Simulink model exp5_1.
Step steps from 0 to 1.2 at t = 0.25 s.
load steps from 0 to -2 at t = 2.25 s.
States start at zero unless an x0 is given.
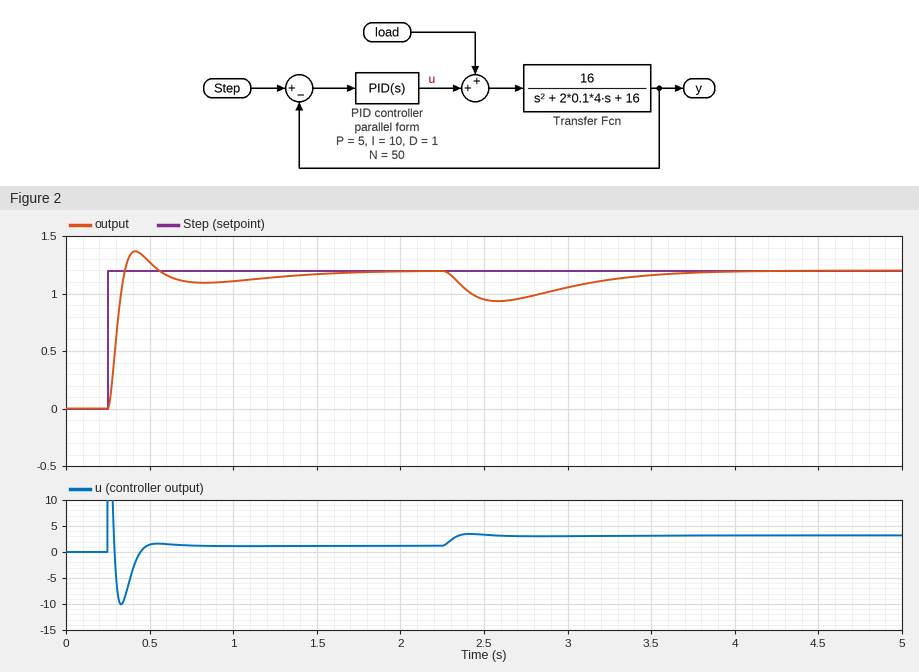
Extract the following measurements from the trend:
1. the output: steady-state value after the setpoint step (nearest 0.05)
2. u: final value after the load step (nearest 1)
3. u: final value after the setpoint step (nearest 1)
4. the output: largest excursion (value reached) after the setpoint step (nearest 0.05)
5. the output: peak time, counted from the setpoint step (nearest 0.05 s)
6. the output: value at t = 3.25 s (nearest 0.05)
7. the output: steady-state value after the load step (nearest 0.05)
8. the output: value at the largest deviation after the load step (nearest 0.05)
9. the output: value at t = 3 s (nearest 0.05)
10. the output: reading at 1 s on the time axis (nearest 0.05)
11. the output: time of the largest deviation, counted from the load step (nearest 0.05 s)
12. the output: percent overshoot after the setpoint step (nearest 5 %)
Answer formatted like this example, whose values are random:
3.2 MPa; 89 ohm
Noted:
1.20; 3; 1; 1.35; 0.15 s; 1.10; 1.20; 0.95; 1.05; 1.10; 0.35 s; 15 %
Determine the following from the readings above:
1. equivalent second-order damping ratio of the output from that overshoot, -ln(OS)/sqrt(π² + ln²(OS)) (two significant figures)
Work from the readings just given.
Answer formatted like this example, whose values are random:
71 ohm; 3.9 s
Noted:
0.52
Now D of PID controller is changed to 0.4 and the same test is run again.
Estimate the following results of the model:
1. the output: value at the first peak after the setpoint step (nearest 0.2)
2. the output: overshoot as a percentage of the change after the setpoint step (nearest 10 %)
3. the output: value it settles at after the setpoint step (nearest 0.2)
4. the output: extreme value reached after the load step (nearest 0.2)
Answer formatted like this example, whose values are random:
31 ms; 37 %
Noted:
1.6; 30 %; 1.2; 0.8
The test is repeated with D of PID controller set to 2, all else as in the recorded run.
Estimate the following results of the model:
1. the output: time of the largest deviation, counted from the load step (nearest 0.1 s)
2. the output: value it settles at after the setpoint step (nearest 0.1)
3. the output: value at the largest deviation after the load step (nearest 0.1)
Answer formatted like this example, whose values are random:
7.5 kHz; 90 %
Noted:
0.5 s; 1.2; 1.0
